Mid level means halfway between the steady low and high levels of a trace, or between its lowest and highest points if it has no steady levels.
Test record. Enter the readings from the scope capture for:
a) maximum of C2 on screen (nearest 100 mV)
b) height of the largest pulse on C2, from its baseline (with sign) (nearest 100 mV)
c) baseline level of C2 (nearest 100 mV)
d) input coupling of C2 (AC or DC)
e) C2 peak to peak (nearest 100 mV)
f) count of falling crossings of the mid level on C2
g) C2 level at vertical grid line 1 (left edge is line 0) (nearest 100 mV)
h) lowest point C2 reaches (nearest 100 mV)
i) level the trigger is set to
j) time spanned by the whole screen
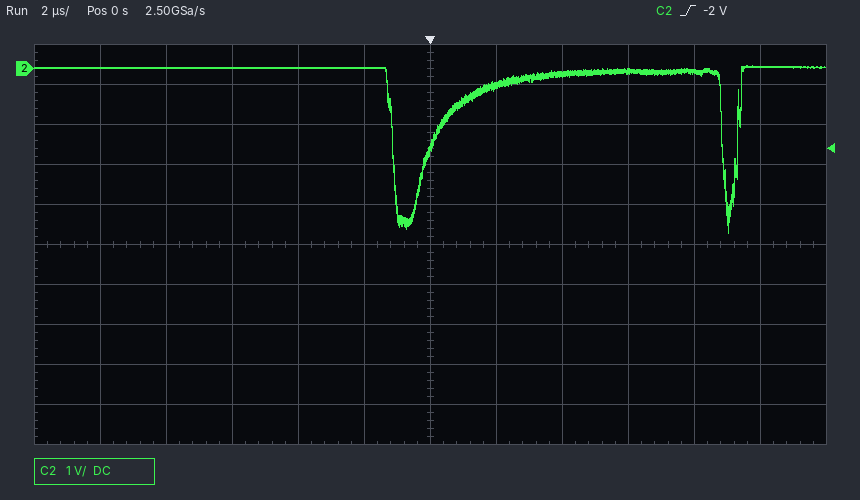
100 mV
-4.1 V
0.0 V
DC
4.2 V
2
0.0 V
-4.1 V
-2 V
24 µs
